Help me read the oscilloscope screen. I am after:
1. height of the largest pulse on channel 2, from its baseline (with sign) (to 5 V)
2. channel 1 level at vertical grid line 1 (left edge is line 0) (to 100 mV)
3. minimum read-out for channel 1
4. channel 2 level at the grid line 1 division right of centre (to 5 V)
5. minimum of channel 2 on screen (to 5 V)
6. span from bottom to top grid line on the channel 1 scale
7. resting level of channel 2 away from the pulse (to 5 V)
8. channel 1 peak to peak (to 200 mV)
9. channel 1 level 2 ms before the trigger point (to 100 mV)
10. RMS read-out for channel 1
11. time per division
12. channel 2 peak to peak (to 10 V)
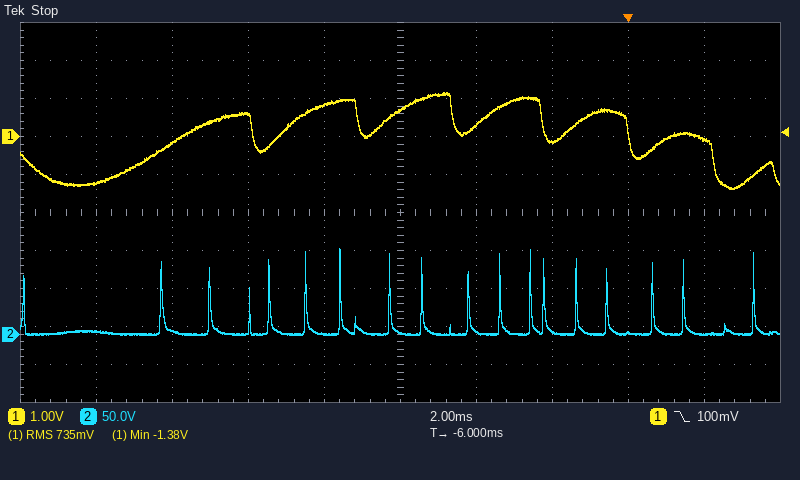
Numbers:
+110 V
-1.2 V
-1.38 V
5 V
0 V
10 V
0 V
2.6 V
-100 mV
735 mV
2 ms
110 V
